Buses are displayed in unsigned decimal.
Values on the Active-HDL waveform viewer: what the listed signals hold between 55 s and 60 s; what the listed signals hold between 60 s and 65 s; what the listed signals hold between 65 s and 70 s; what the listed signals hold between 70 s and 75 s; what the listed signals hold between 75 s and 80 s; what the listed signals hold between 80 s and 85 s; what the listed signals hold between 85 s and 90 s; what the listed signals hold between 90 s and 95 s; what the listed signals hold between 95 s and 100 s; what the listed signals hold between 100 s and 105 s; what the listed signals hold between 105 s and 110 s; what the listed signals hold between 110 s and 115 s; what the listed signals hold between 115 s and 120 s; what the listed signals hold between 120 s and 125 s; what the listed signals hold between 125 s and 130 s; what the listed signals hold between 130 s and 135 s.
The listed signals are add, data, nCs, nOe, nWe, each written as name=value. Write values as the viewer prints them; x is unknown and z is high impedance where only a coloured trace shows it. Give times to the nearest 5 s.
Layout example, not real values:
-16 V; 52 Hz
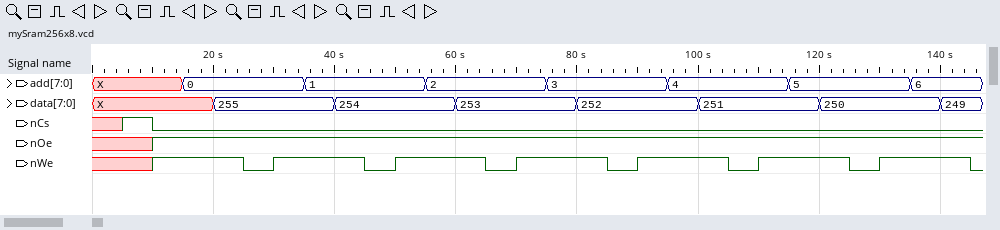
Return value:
add=2, data=254, nCs=0, nOe=1, nWe=1; add=2, data=253, nCs=0, nOe=1, nWe=1; add=2, data=253, nCs=0, nOe=1, nWe=0; add=2, data=253, nCs=0, nOe=1, nWe=1; add=3, data=253, nCs=0, nOe=1, nWe=1; add=3, data=252, nCs=0, nOe=1, nWe=1; add=3, data=252, nCs=0, nOe=1, nWe=0; add=3, data=252, nCs=0, nOe=1, nWe=1; add=4, data=252, nCs=0, nOe=1, nWe=1; add=4, data=251, nCs=0, nOe=1, nWe=1; add=4, data=251, nCs=0, nOe=1, nWe=0; add=4, data=251, nCs=0, nOe=1, nWe=1; add=5, data=251, nCs=0, nOe=1, nWe=1; add=5, data=250, nCs=0, nOe=1, nWe=1; add=5, data=250, nCs=0, nOe=1, nWe=0; add=5, data=250, nCs=0, nOe=1, nWe=1
